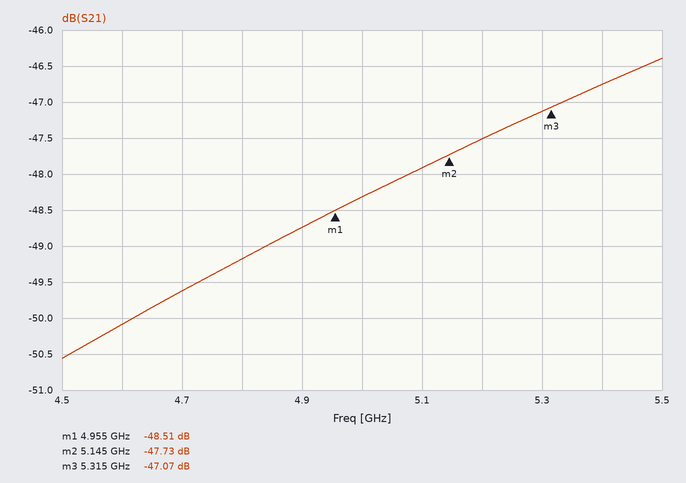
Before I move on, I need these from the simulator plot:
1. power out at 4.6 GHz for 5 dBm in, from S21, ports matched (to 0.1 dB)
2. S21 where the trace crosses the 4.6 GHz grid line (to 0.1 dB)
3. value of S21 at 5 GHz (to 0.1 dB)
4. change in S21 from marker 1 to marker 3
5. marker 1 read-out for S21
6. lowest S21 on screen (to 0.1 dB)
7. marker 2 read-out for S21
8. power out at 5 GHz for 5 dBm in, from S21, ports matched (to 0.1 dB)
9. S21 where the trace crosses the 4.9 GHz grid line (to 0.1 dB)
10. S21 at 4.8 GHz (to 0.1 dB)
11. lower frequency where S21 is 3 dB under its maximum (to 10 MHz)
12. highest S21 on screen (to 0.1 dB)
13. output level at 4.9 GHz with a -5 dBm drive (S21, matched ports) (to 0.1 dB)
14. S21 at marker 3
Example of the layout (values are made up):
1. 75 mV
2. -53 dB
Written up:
1. -45.1 dBm
2. -50.1 dB
3. -48.3 dB
4. 1.44 dB
5. -48.51 dB
6. -50.6 dB
7. -47.73 dB
8. -43.3 dBm
9. -48.7 dB
10. -49.2 dB
11. 4.75 GHz
12. -46.4 dB
13. -53.7 dBm
14. -47.07 dB
